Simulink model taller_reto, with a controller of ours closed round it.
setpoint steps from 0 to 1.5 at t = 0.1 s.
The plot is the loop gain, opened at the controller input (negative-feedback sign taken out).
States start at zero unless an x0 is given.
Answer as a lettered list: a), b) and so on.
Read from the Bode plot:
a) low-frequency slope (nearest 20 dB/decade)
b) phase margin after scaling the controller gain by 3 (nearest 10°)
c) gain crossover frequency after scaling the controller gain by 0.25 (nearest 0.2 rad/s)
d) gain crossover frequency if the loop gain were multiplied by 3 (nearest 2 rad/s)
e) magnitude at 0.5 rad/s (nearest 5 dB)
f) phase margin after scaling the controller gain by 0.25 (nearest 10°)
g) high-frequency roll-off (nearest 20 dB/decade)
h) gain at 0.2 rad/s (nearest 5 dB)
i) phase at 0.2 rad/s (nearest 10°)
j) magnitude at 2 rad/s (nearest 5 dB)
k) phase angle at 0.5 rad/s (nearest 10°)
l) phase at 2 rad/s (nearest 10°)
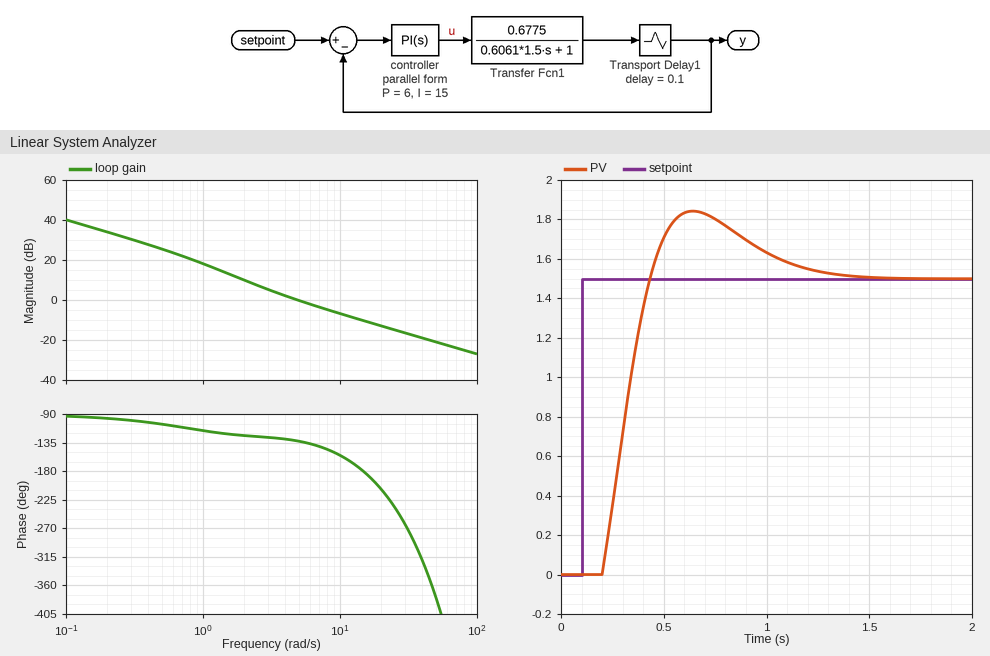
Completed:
a) -20 dB/decade
b) 10°
c) 1.6 rad/s
d) 14 rad/s
e) 25 dB
f) 60°
g) -20 dB/decade
h) 35 dB
i) -100°
j) 10 dB
k) -110°
l) -120°
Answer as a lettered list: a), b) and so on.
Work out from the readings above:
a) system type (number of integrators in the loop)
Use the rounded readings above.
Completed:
a) 1
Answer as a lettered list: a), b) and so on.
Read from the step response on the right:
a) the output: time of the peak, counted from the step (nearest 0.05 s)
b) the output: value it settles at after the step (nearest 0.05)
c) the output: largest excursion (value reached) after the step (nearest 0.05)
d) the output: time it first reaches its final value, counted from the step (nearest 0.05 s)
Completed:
a) 0.55 s
b) 1.50
c) 1.85
d) 0.35 s
